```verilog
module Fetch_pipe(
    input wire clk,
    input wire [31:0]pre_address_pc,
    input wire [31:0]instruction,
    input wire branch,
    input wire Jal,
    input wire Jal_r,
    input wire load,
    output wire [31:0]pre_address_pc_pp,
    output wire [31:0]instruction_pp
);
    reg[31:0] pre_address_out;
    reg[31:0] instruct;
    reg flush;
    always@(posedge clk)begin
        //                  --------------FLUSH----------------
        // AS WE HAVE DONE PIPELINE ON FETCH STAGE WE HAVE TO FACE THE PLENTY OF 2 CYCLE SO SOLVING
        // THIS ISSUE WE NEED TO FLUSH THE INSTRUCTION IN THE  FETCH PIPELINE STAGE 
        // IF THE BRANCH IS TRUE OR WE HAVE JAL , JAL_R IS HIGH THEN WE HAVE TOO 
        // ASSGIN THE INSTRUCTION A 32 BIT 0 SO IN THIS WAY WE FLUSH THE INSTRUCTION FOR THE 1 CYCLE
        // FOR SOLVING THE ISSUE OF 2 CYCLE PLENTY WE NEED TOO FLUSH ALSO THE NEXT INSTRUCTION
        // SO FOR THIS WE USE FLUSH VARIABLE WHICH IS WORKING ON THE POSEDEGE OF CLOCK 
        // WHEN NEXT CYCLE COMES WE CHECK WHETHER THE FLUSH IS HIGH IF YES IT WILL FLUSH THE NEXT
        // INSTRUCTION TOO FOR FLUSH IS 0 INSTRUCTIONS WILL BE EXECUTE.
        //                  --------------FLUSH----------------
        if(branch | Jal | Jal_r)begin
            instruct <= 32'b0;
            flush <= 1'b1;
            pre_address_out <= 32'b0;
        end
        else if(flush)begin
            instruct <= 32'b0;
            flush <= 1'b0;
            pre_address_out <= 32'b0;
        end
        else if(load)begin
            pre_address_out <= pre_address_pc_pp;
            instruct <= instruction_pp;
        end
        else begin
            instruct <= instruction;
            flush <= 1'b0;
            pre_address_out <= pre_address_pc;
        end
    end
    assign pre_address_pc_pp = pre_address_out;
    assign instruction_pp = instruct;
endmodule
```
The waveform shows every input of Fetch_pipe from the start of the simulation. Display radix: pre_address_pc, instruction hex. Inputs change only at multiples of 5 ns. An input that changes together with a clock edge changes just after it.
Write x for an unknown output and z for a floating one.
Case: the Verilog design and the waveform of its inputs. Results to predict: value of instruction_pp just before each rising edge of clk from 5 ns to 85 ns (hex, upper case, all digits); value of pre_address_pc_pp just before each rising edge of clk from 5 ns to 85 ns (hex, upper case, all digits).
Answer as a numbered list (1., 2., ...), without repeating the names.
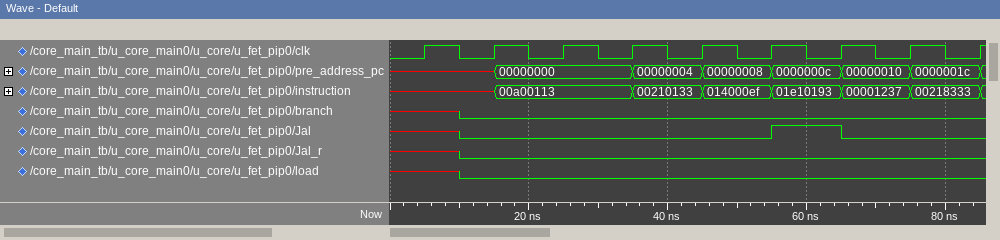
1. x, x, x, 00A00113, 00A00113, 00210133, 014000EF, 00000000, 00000000
2. x, x, x, 00000000, 00000000, 00000004, 00000008, 00000000, 00000000
